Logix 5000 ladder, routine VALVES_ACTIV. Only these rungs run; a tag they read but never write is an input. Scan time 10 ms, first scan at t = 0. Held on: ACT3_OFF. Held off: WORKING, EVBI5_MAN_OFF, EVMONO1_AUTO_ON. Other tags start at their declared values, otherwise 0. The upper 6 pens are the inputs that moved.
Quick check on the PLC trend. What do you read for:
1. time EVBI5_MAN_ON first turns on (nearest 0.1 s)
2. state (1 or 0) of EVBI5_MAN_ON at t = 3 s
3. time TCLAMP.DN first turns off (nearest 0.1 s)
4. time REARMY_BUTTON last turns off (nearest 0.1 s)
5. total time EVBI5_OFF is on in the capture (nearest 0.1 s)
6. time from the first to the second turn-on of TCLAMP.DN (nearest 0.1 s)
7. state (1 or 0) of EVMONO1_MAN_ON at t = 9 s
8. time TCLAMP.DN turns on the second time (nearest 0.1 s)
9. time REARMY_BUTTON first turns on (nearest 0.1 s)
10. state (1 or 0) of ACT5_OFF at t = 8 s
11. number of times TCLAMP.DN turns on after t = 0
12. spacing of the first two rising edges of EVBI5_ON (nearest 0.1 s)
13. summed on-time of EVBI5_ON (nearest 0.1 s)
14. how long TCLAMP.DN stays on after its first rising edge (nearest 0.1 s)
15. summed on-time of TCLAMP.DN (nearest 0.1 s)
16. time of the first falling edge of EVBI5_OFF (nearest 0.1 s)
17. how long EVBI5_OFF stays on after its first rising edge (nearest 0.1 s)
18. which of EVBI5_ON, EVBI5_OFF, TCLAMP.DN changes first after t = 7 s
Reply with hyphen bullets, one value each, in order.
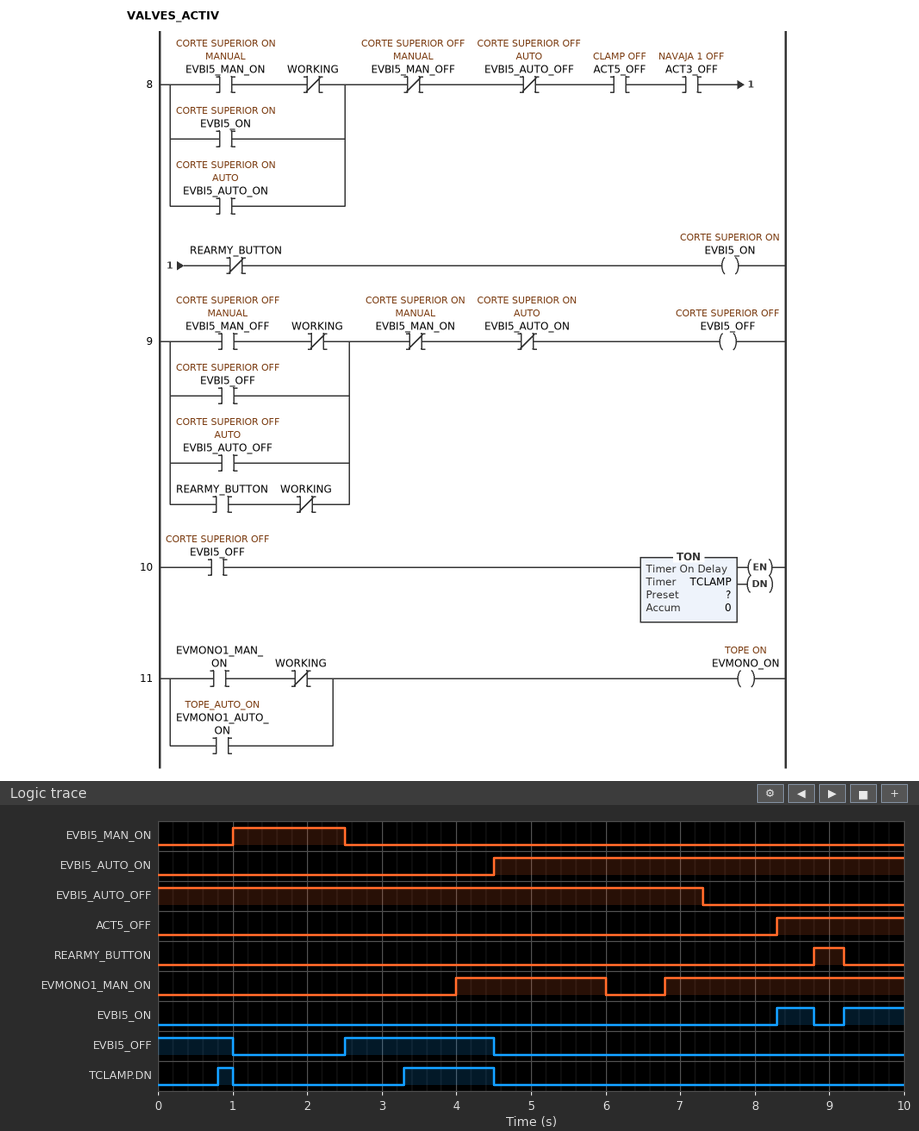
- 1.0 s
- 0
- 1.0 s
- 9.2 s
- 3.0 s
- 2.5 s
- 1
- 3.3 s
- 8.8 s
- 0
- 2
- 0.9 s
- 1.3 s
- 0.2 s
- 1.4 s
- 1.0 s
- 2.0 s
- EVBI5_ON
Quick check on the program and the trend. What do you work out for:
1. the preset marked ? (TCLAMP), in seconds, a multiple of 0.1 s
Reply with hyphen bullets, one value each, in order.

- 0.8 s
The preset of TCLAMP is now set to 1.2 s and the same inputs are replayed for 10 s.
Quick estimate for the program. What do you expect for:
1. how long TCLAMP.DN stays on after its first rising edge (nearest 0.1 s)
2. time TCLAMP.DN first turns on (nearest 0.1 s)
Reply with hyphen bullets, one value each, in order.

- 0.8 s
- 3.7 s
